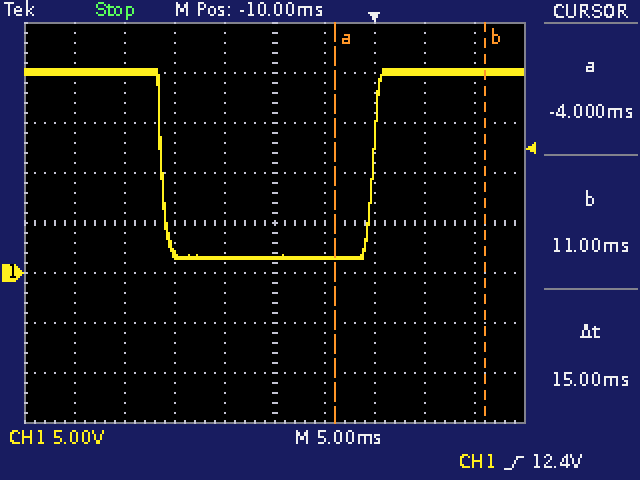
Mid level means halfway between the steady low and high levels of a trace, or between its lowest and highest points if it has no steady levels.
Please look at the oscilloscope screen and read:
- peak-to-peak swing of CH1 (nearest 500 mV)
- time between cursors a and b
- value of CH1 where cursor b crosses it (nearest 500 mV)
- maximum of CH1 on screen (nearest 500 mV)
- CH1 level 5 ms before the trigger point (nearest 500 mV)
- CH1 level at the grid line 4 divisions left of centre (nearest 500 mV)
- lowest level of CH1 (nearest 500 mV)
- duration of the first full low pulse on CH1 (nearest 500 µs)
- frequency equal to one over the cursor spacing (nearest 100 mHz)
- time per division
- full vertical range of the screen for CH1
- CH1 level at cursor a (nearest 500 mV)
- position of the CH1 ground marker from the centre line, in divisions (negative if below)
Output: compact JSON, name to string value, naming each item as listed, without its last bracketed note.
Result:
{"peak-to-peak swing of CH1": "19.0 V", "time between cursors a and b": "15 ms", "value of CH1 where cursor b crosses it": "20.0 V", "maximum of CH1 on screen": "20.5 V", "CH1 level 5 ms before the trigger point": "1.5 V", "CH1 level at the grid line 4 divisions left of centre": "20.0 V", "lowest level of CH1": "1.5 V", "duration of the first full low pulse on CH1": "21.0 ms", "frequency equal to one over the cursor spacing": "66.7 Hz", "time per division": "5 ms", "full vertical range of the screen for CH1": "40 V", "CH1 level at cursor a": "1.5 V", "position of the CH1 ground marker from the centre line, in divisions": "-1.0 div"}
